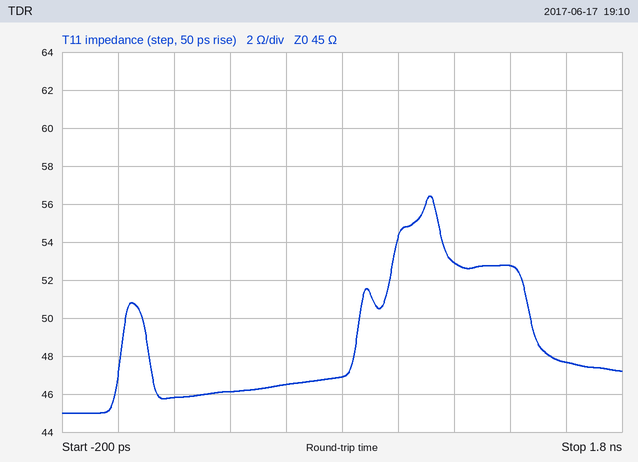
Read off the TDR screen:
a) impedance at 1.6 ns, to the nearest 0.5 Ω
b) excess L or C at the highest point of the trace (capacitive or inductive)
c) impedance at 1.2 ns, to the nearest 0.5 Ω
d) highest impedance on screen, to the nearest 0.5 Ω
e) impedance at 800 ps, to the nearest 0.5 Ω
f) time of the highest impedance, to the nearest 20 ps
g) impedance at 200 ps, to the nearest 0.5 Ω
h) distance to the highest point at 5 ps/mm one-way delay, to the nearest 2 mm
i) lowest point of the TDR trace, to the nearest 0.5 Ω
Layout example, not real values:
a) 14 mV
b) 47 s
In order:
a) 47.5 Ω
b) inductive
c) 53.0 Ω
d) 56.5 Ω
e) 47.0 Ω
f) 1.12 ns
g) 46.0 Ω
h) 112 mm
i) 45.0 Ω
